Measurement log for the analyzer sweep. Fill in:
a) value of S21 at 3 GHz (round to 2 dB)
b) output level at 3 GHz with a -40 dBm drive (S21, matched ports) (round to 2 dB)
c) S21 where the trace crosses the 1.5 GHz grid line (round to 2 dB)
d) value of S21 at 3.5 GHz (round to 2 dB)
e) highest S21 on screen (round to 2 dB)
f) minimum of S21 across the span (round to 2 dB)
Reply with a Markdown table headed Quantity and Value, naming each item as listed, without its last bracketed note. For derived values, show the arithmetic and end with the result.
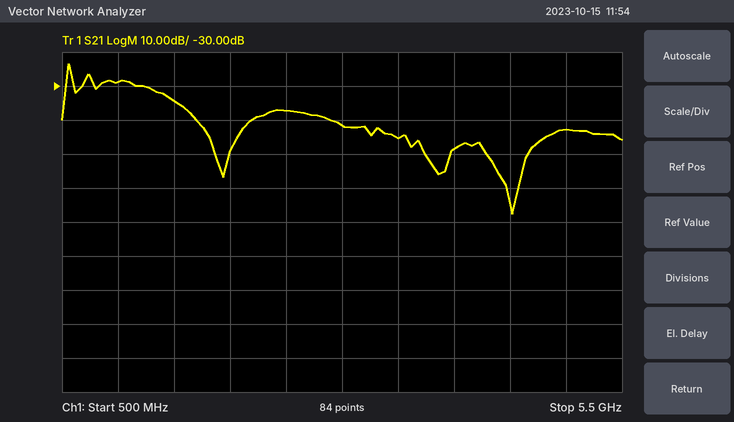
| Quantity | Value |
|---|---|
| value of S21 at 3 GHz | -42 dB |
| output level at 3 GHz with a -40 dBm drive (S21, matched ports) | -40 dBm + (-42 dB) = -82 dBm |
| S21 where the trace crosses the 1.5 GHz grid line | -34 dB |
| value of S21 at 3.5 GHz | -46 dB |
| highest S21 on screen | -24 dB |
| minimum of S21 across the span | -68 dB |
